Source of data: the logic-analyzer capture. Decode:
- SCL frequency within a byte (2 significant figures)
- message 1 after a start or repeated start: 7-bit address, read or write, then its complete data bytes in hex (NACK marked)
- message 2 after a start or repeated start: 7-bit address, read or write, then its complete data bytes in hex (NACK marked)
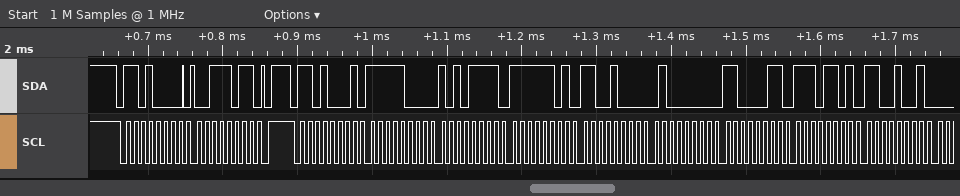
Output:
100 kHz
0x68 write: 3B
0x68 read: F8 AF FD C8 40 C3 ED C9
